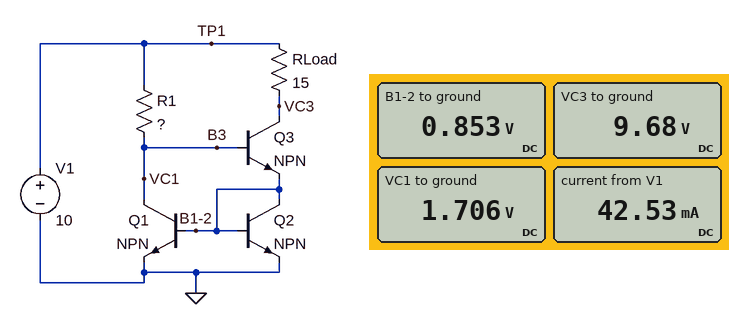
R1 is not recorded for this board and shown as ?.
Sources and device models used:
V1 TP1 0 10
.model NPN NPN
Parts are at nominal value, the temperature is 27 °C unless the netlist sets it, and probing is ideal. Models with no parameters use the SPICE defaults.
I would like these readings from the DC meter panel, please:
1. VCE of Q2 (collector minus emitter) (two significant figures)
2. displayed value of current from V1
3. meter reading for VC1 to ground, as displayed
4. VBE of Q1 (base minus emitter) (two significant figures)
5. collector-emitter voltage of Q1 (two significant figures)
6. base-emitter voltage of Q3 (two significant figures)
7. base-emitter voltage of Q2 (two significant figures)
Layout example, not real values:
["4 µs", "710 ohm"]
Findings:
["850 mV", "42.53 mA", "1.706 V", "850 mV", "1.7 V", "850 mV", "850 mV"]
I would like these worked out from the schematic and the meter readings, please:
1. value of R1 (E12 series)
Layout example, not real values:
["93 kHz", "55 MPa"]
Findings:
["390 Ω"]
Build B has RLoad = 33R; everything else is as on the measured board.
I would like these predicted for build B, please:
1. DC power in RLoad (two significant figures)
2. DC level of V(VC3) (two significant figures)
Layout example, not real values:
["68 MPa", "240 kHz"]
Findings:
["15 mW", "9.3 V"]
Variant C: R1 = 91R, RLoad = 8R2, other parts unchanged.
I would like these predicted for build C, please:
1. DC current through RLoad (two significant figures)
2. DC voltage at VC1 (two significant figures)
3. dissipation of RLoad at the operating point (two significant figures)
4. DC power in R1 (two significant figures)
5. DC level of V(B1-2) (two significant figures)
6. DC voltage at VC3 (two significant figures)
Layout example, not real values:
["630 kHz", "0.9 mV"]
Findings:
["90 mA", "1.8 V", "67 mW", "740 mW", "890 mV", "9.3 V"]
